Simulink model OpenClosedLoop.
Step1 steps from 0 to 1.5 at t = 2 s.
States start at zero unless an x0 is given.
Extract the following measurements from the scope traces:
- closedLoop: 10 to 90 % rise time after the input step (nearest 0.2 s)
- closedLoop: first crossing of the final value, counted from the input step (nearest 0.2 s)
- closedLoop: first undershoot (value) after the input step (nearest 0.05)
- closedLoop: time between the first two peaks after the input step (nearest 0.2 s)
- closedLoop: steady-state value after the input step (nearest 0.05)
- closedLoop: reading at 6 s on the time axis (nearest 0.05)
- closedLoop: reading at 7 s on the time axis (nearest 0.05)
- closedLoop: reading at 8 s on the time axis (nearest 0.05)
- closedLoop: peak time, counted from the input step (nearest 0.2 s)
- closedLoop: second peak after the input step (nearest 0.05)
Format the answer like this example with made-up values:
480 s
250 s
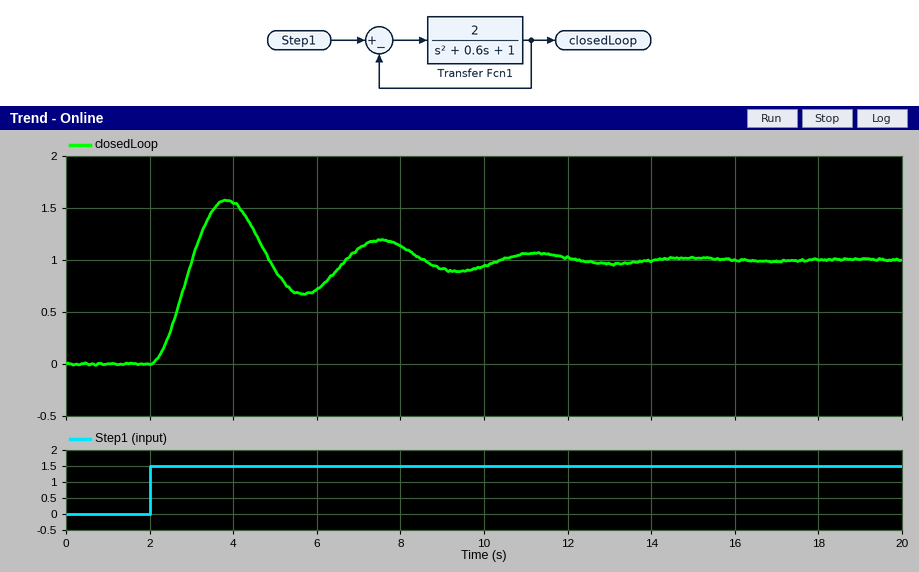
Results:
0.6 s
1.0 s
0.65
3.6 s
1.00
0.70
1.10
1.15
1.8 s
1.20
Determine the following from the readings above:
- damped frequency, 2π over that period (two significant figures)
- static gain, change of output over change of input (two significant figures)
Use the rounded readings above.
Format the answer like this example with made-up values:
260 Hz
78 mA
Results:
1.7 rad/s
0.67
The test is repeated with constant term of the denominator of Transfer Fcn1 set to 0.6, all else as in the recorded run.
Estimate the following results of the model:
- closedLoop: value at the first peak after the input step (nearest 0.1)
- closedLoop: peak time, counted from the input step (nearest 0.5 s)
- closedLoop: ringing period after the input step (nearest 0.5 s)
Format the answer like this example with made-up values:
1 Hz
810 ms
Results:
1.8
2.0 s
4.0 s
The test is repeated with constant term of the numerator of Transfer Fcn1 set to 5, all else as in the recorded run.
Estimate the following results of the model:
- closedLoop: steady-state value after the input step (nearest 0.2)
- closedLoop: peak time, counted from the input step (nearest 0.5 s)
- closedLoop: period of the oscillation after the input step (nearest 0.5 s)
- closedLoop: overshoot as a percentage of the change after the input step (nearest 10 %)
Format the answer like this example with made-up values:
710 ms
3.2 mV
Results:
1.2
1.5 s
2.5 s
70 %
